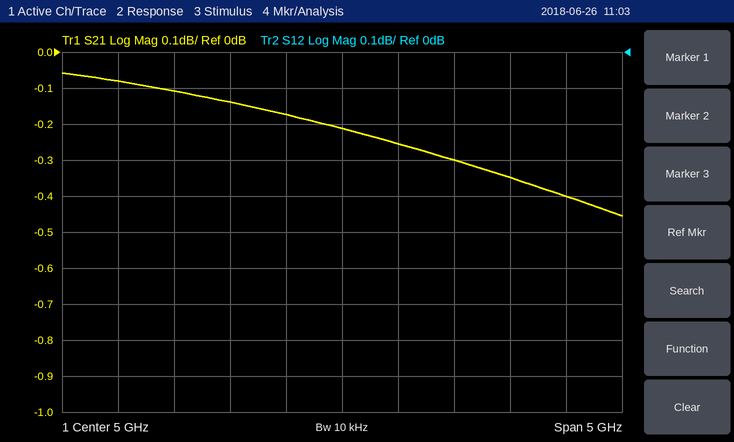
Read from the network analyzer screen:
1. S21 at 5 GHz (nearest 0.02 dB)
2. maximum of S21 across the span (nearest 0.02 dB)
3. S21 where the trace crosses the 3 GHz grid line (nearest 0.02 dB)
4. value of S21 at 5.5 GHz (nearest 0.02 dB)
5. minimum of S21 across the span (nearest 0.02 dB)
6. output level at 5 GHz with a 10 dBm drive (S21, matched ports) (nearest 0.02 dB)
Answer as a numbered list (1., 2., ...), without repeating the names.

1. -0.22 dB
2. -0.06 dB
3. -0.08 dB
4. -0.26 dB
5. -0.46 dB
6. 9.78 dBm
